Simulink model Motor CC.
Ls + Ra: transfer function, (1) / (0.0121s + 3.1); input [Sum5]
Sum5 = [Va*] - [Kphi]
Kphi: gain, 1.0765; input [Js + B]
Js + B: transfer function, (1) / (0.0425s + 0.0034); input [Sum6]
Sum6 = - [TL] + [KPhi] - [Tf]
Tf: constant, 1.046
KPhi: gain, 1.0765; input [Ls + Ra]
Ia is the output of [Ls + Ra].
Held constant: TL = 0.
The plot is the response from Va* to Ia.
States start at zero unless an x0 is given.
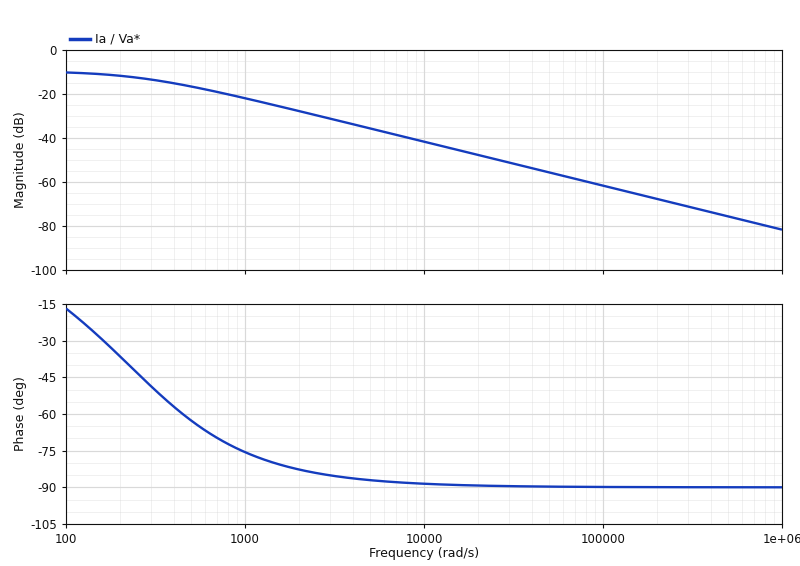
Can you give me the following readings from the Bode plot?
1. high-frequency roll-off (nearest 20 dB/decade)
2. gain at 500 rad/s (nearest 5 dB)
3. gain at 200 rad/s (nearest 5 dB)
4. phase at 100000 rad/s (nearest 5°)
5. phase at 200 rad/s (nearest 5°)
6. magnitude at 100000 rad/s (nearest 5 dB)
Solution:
-20 dB/decade
-15 dB
-10 dB
-90°
-35°
-60 dB
